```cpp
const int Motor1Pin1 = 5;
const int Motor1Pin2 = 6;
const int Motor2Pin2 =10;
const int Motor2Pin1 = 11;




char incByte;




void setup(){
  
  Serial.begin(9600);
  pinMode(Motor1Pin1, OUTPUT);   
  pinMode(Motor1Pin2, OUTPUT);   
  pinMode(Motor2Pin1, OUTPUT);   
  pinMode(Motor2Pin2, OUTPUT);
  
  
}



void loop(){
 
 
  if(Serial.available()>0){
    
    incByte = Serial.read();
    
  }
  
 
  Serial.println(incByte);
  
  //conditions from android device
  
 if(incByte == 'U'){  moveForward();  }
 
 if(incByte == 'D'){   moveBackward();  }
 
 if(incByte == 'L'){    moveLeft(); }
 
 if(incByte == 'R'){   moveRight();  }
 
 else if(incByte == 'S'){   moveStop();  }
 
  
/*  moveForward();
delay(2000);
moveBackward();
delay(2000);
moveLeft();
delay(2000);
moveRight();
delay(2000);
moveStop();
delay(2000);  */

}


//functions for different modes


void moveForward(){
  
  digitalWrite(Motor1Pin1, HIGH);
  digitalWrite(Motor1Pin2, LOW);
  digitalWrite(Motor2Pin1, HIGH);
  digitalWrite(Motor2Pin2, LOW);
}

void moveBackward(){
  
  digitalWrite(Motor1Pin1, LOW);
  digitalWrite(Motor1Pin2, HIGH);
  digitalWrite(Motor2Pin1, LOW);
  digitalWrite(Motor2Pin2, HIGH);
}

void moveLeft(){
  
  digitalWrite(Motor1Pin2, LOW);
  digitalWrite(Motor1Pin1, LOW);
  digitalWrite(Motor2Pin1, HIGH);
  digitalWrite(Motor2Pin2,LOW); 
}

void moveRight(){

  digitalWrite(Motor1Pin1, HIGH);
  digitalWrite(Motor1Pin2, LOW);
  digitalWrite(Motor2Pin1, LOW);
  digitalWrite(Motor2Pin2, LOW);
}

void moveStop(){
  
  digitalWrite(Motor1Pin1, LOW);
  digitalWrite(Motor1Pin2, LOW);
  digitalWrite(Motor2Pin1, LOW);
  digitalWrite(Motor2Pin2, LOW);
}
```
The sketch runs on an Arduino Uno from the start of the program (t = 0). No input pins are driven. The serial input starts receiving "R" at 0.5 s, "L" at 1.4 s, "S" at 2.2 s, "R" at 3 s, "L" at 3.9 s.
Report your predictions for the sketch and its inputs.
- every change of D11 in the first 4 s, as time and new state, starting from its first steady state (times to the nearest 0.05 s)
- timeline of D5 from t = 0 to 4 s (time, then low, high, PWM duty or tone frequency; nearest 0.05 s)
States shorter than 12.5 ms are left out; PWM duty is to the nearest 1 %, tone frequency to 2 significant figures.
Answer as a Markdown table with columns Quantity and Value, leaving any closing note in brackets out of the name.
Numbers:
| Quantity | Value |
|---|---|
| every change of D11 in the first 4 s, as time and new state, starting from its first steady state | 0 s low; 1.4 s high; 2.2 s low; 3.9 s high |
| timeline of D5 from t = 0 to 4 s | 0 s low; 0.5 s high; 1.4 s low; 3 s high; 3.9 s low |
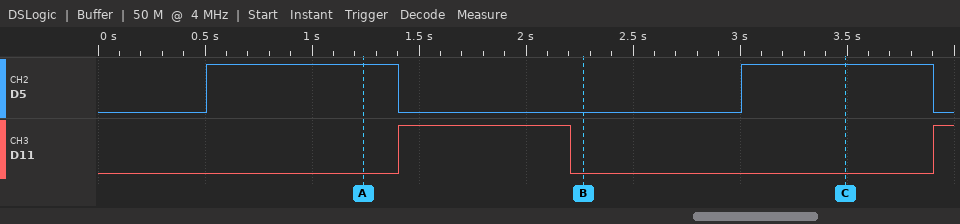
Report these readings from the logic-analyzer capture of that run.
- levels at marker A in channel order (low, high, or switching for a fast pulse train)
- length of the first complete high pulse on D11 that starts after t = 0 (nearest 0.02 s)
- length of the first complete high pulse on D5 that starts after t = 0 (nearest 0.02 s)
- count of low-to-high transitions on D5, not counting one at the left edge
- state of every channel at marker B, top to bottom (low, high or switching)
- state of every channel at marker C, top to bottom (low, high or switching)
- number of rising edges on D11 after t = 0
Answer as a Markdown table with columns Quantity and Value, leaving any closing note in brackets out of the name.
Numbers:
| Quantity | Value |
|---|---|
| levels at marker A in channel order | D5 high, D11 low |
| length of the first complete high pulse on D11 that starts after t = 0 | 0.80 s |
| length of the first complete high pulse on D5 that starts after t = 0 | 0.90 s |
| count of low-to-high transitions on D5, not counting one at the left edge | 2 |
| state of every channel at marker B, top to bottom | D5 low, D11 low |
| state of every channel at marker C, top to bottom | D5 high, D11 low |
| number of rising edges on D11 after t = 0 | 2 |
